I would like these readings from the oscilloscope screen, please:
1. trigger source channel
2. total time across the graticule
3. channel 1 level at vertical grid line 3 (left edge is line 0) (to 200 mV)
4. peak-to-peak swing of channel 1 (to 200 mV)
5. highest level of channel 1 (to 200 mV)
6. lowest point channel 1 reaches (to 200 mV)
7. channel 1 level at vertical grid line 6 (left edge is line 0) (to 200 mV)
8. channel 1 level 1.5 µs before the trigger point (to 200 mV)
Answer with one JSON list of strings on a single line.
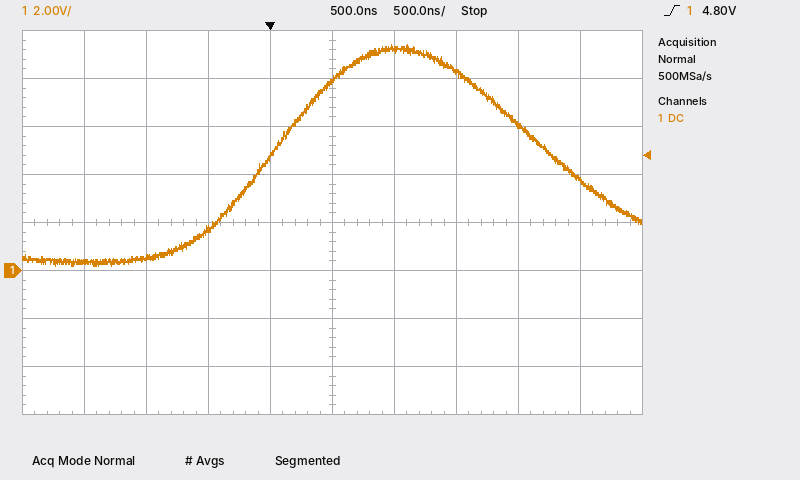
["channel 1", "5 µs", "1.6 V", "9.2 V", "9.4 V", "200 mV", "9.2 V", "400 mV"]
